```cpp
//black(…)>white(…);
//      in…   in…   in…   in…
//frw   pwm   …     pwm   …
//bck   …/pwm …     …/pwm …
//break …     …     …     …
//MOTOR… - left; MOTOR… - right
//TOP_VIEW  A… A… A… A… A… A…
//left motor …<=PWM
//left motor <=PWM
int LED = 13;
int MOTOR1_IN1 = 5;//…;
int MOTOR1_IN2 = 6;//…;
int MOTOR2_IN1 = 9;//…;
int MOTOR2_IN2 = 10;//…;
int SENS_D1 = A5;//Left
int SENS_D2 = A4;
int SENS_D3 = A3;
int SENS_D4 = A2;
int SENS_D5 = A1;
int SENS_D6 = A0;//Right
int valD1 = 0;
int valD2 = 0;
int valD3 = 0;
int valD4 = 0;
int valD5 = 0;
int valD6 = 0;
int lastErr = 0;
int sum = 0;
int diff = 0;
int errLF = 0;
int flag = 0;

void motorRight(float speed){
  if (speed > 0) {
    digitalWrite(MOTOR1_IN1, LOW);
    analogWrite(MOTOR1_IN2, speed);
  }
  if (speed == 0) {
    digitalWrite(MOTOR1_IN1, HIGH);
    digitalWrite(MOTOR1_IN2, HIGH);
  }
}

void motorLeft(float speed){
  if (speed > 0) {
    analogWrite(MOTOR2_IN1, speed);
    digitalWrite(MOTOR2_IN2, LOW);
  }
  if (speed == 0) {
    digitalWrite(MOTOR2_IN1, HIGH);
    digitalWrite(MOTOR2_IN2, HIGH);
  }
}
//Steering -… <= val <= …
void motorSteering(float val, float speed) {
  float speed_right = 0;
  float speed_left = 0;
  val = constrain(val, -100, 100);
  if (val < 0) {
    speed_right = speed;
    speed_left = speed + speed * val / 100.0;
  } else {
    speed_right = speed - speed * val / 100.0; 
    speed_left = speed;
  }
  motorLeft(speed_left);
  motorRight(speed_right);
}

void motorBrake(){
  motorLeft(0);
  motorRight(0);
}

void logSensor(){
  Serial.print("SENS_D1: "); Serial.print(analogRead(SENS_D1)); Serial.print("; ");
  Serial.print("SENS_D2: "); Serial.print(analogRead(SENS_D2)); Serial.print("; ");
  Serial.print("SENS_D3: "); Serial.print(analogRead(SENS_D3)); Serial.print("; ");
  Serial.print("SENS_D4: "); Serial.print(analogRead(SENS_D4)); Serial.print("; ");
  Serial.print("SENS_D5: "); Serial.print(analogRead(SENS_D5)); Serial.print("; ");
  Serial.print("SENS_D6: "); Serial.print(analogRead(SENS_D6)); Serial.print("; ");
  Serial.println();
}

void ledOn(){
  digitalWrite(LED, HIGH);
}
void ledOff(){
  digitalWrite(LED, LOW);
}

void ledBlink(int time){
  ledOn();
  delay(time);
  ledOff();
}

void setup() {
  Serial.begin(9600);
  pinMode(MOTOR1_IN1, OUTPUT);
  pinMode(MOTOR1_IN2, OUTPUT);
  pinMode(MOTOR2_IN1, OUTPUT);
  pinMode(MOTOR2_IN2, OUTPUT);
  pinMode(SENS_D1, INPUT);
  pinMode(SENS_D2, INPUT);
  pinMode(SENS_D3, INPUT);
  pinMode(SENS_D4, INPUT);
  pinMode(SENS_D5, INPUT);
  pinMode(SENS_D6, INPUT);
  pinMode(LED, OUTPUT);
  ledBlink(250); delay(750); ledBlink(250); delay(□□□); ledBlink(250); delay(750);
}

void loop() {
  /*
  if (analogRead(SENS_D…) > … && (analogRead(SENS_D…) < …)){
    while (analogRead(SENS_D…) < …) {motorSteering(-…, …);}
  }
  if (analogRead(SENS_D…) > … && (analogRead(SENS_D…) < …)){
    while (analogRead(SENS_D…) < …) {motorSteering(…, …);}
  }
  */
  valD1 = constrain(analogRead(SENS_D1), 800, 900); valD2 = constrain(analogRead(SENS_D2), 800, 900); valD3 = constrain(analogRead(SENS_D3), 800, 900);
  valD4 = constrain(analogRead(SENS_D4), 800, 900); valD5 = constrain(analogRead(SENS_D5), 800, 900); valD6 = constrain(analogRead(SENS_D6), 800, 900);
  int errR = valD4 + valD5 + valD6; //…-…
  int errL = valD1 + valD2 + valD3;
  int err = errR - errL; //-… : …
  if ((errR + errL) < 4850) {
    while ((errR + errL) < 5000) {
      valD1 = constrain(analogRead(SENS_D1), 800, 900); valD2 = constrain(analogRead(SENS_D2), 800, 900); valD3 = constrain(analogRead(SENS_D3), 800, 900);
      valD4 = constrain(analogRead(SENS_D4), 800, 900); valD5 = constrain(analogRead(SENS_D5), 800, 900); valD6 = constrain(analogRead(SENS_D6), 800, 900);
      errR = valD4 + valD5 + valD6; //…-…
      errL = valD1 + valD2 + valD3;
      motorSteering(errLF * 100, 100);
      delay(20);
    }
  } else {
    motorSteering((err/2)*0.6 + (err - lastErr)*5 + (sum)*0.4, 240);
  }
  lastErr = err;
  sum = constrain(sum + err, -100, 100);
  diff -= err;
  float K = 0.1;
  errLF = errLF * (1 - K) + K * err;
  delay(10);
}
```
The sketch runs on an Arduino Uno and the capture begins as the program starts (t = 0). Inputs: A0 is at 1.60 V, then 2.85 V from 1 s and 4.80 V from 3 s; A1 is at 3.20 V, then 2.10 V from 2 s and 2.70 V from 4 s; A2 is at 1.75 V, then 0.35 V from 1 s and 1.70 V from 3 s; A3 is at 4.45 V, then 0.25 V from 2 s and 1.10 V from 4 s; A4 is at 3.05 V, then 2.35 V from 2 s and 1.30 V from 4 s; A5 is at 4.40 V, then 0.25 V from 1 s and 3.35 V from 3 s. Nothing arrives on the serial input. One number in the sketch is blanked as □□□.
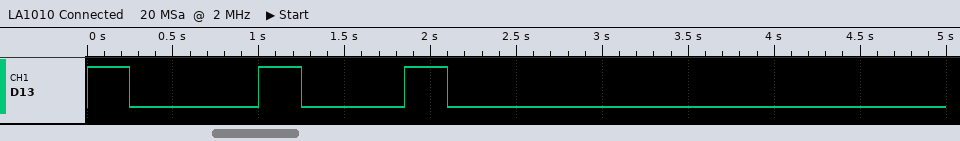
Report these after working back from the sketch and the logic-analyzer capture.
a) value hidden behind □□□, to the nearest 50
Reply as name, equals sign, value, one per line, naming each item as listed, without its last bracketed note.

value hidden behind □□□, to the nearest 50 = 600
